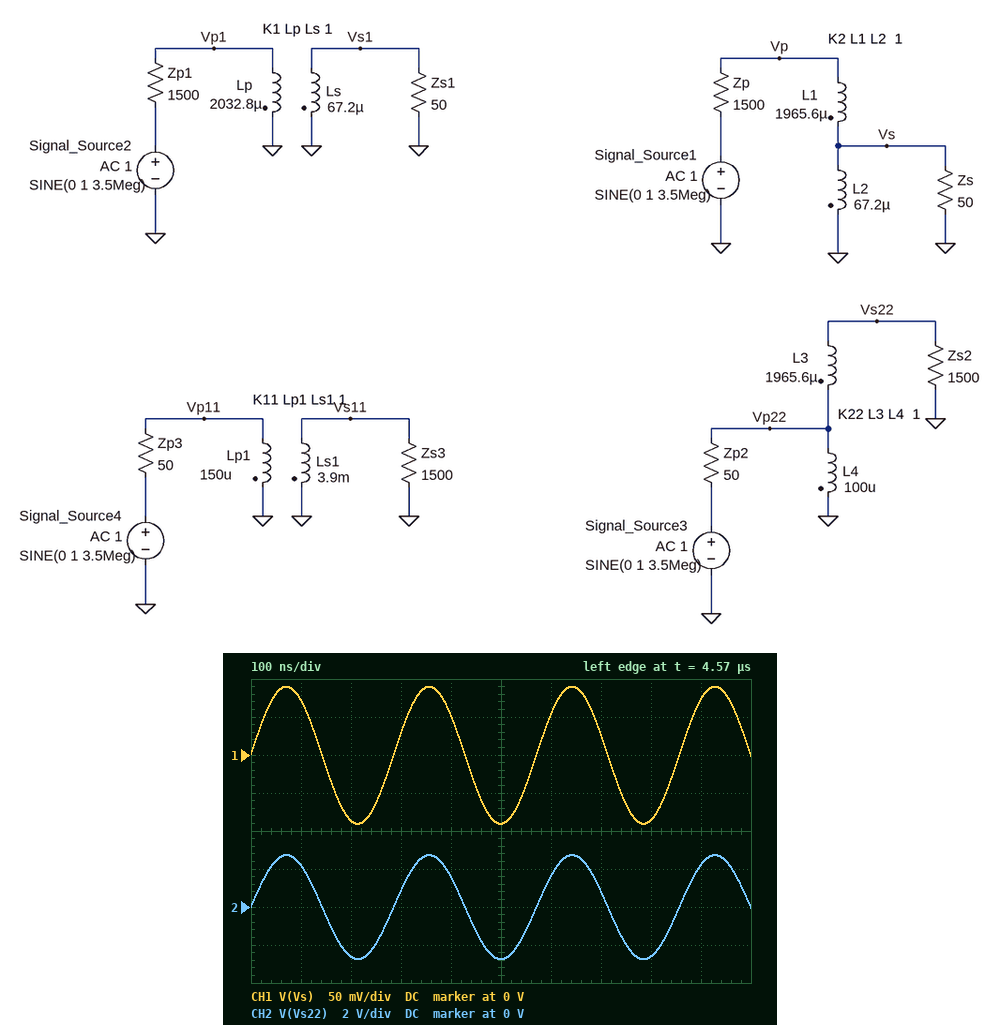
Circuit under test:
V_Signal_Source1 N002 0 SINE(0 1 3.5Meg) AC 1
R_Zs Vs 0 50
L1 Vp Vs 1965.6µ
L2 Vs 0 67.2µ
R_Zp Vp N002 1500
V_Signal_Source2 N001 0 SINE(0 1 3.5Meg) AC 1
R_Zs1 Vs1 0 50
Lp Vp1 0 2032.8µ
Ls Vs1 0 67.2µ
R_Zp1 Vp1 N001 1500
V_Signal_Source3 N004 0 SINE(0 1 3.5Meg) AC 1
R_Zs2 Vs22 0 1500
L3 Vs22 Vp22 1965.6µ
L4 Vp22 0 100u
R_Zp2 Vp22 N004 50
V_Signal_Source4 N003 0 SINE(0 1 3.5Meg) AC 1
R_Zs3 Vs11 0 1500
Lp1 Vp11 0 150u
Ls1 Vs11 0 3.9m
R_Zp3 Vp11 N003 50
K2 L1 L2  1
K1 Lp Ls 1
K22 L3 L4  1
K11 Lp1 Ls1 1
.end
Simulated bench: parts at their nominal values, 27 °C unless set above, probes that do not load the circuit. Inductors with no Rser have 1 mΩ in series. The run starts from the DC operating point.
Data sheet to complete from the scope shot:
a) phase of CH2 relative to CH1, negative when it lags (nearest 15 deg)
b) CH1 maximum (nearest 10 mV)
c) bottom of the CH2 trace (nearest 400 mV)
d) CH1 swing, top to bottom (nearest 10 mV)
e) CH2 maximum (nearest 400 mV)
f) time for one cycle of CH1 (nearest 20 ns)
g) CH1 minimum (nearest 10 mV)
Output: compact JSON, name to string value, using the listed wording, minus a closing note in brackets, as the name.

{"phase of CH2 relative to CH1, negative when it lags": "0 deg", "CH1 maximum": "90 mV", "bottom of the CH2 trace": "-2.8 V", "CH1 swing, top to bottom": "180 mV", "CH2 maximum": "2.8 V", "time for one cycle of CH1": "280 ns", "CH1 minimum": "-90 mV"}
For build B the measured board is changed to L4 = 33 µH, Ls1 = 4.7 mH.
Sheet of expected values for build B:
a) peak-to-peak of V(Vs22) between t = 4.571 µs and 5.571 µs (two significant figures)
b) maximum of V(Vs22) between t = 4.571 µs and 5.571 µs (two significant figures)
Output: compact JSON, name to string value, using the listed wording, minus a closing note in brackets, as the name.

{"peak-to-peak of V(Vs22) between t = 4.571 µs and 5.571 µs": "4.9 V", "maximum of V(Vs22) between t = 4.571 µs and 5.571 µs": "2.5 V"}
